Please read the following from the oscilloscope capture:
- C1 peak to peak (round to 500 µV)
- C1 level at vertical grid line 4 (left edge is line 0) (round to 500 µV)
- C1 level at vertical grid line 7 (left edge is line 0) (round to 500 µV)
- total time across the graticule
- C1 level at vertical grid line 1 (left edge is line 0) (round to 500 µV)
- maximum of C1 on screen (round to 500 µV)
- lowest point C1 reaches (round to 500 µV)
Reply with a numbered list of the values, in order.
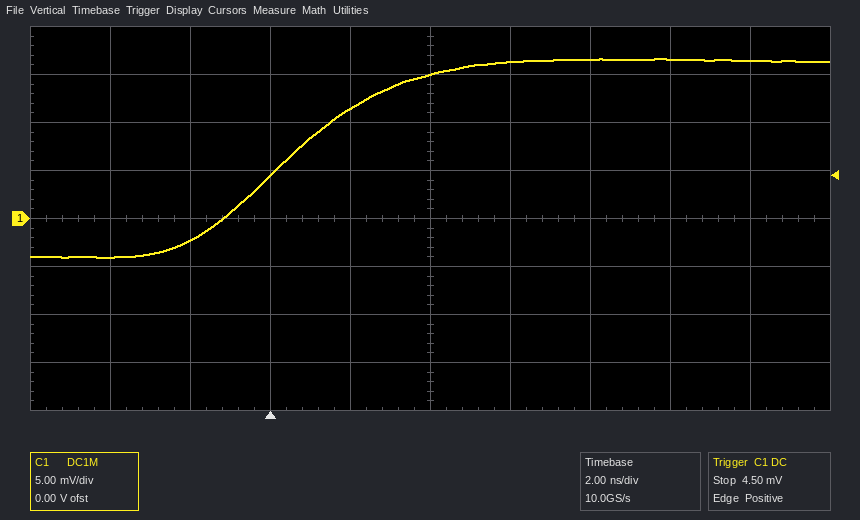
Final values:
1. 20.5 mV
2. 11.5 mV
3. 16.5 mV
4. 20 ns
5. -4.0 mV
6. 16.5 mV
7. -4.0 mV
